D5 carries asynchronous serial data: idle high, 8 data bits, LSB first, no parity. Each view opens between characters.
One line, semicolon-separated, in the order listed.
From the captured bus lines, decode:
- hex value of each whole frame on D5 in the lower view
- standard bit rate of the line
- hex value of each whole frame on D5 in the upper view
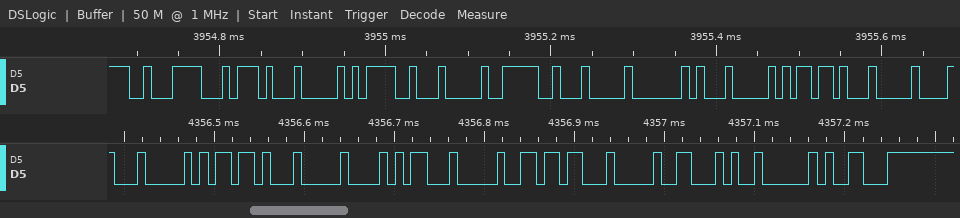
04, 6D, 04, A8, 04, B6, 04, 46, 02, 19; 115200 baud; E2, 74, 04, 3D, 04, 3E, 04, 40, 04, 6D, 04
